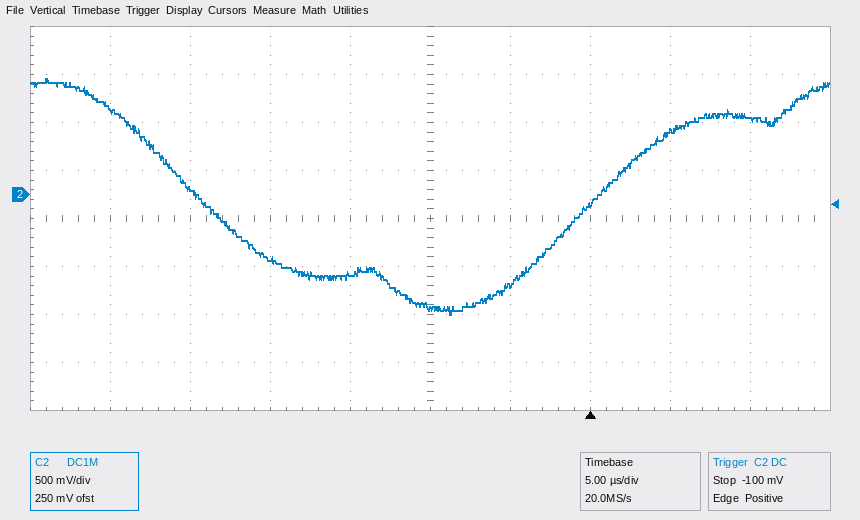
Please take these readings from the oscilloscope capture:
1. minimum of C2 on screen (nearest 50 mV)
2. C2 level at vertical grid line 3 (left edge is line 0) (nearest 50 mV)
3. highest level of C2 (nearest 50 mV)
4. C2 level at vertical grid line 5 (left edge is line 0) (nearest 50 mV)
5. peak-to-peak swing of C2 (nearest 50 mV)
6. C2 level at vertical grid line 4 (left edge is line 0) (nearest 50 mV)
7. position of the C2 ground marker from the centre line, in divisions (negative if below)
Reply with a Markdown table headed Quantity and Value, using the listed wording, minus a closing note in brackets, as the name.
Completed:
| Quantity | Value |
|---|---|
| minimum of C2 on screen | -1.25 V |
| C2 level at vertical grid line 3 (left edge is line 0) | -700 mV |
| highest level of C2 | 1.20 V |
| C2 level at vertical grid line 5 (left edge is line 0) | -1.15 V |
| peak-to-peak swing of C2 | 2.45 V |
| C2 level at vertical grid line 4 (left edge is line 0) | -850 mV |
| position of the C2 ground marker from the centre line, in divisions | +0.5 div |
